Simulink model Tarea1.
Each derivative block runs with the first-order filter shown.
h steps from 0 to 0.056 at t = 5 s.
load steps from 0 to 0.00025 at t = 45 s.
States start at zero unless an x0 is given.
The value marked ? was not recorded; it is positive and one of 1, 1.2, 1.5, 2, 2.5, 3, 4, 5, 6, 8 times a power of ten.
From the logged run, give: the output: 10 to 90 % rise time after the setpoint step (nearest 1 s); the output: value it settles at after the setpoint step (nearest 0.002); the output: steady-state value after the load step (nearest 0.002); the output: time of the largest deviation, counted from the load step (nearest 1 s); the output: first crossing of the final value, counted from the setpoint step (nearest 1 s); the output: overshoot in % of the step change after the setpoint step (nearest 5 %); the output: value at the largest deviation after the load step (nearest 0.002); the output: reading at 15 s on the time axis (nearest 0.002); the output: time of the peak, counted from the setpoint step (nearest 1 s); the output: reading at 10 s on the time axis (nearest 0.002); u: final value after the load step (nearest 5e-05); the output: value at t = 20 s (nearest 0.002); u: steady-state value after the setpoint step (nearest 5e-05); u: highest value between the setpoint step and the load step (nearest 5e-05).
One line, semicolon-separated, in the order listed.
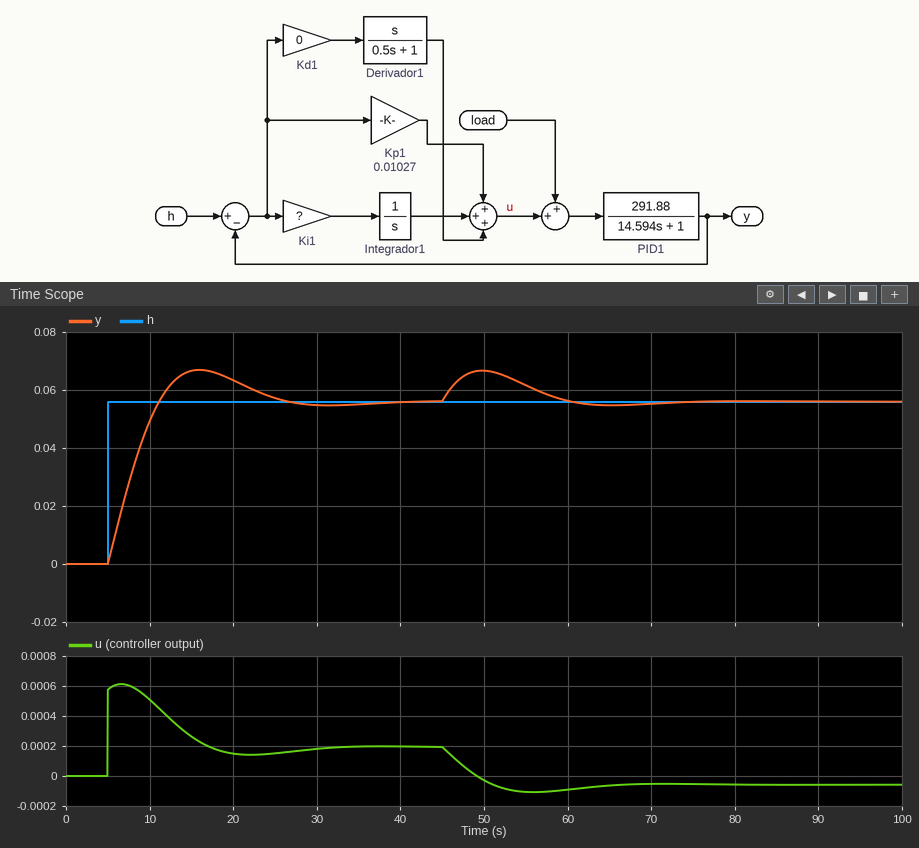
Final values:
5 s; 0.056; 0.056; 5 s; 6 s; 20 %; 0.066; 0.066; 11 s; 0.050; -0.00005; 0.064; 0.00020; 0.00060
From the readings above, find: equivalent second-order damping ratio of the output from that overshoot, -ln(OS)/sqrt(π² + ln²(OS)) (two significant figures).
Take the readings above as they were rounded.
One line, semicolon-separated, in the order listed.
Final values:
0.46
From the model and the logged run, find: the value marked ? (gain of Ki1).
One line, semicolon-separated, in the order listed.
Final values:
0.003
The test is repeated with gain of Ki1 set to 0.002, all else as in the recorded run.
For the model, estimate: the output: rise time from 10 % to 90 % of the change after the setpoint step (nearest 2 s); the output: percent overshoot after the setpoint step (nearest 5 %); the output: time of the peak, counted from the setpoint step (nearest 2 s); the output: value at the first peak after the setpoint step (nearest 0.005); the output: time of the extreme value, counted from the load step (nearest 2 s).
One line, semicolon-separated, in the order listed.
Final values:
6 s; 15 %; 14 s; 0.065; 6 s
